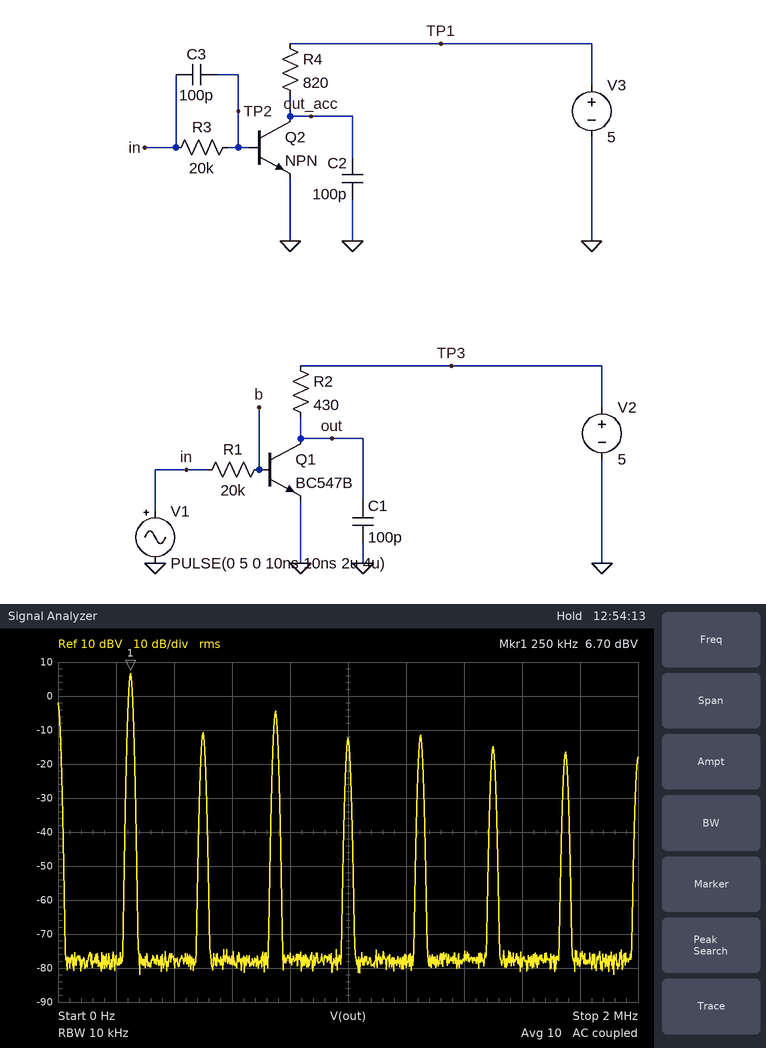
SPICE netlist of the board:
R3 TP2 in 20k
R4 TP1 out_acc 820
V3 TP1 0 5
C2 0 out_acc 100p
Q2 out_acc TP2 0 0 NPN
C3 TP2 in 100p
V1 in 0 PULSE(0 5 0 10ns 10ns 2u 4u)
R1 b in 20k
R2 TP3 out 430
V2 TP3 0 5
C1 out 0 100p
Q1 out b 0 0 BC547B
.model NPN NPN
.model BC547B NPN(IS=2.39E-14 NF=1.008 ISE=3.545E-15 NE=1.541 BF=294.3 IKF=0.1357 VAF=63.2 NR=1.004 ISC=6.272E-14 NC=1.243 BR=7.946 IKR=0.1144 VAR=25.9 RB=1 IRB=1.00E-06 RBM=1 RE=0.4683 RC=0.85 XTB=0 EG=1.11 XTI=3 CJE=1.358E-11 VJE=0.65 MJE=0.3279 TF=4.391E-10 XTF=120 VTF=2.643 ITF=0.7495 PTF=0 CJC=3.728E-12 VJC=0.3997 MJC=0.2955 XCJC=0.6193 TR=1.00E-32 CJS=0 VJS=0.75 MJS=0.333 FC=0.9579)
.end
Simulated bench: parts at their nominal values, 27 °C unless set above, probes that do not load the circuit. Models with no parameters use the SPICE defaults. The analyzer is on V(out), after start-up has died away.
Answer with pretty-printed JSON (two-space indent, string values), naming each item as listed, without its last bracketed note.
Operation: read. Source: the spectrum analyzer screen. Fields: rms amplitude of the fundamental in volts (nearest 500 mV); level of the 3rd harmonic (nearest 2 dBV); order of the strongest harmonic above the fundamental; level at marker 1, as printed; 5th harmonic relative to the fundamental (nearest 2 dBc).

{
  "rms amplitude of the fundamental in volts": "2.0 V",
  "level of the 3rd harmonic": "-4 dBV",
  "order of the strongest harmonic above the fundamental": "3",
  "level at marker 1, as printed": "6.70 dBV",
  "5th harmonic relative to the fundamental": "-18 dBc"
}
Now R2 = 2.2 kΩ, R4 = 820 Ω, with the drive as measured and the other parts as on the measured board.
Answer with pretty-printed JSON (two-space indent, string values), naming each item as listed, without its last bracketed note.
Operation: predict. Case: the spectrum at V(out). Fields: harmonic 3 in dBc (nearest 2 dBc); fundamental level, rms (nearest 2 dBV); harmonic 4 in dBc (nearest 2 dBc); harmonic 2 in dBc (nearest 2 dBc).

{
  "harmonic 3 in dBc": "-14 dBc",
  "fundamental level, rms": "6 dBV",
  "harmonic 4 in dBc": "-16 dBc",
  "harmonic 2 in dBc": "-12 dBc"
}
